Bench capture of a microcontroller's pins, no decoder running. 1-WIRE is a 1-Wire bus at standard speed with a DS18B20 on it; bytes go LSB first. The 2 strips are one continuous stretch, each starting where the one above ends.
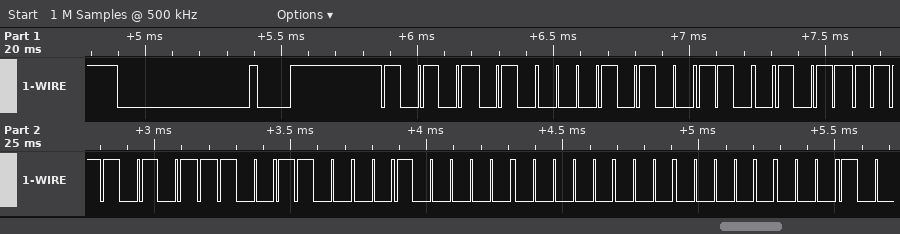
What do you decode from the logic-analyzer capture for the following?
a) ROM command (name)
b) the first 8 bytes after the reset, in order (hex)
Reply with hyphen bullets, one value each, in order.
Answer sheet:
- Match ROM
- 55 28 D3 AF 33 04 00 00
